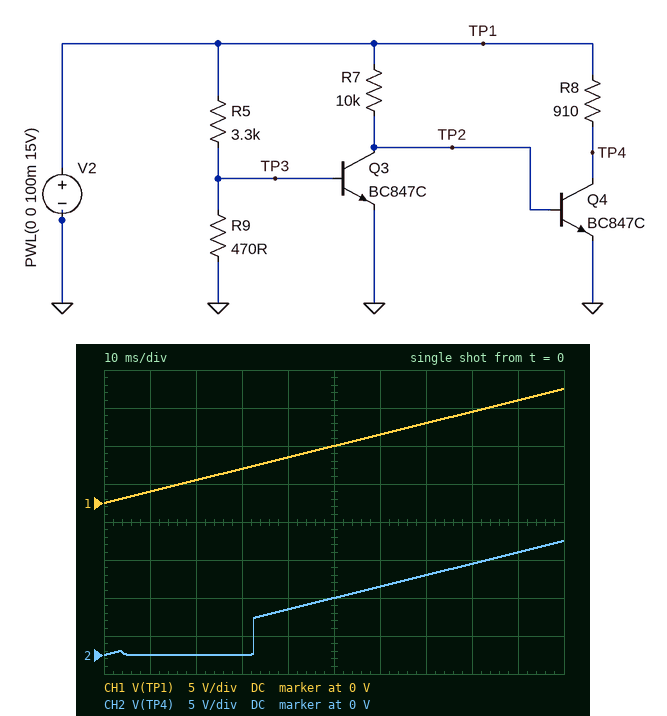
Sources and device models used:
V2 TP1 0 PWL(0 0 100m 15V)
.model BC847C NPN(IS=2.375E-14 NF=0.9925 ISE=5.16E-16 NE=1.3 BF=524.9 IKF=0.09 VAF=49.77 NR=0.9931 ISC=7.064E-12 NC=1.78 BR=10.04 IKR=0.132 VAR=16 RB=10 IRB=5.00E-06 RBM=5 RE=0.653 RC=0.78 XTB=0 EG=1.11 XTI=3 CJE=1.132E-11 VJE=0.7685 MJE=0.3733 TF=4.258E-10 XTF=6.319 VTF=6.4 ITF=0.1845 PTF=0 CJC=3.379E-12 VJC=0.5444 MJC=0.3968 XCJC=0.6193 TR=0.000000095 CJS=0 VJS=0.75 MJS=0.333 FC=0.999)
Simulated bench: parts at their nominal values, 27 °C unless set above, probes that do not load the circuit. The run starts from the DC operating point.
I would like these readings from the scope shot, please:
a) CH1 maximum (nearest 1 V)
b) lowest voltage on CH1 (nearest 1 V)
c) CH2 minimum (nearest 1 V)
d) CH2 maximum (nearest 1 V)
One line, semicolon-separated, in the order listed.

15 V; 0 V; 0 V; 15 V
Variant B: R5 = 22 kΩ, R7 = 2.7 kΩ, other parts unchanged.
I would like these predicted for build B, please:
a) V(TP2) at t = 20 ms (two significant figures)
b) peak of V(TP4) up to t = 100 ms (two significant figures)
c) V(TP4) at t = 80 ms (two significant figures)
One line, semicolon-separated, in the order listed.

700 mV; 510 mV; 36 mV
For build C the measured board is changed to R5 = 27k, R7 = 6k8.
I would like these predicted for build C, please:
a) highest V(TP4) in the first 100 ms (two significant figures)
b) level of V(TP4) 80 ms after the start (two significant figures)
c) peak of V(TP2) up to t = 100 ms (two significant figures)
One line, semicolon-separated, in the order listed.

510 mV; 42 mV; 750 mV
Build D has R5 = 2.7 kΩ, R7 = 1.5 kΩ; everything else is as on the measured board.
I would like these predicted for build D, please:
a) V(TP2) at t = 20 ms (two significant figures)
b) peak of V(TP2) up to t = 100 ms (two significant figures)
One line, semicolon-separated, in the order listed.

720 mV; 730 mV
